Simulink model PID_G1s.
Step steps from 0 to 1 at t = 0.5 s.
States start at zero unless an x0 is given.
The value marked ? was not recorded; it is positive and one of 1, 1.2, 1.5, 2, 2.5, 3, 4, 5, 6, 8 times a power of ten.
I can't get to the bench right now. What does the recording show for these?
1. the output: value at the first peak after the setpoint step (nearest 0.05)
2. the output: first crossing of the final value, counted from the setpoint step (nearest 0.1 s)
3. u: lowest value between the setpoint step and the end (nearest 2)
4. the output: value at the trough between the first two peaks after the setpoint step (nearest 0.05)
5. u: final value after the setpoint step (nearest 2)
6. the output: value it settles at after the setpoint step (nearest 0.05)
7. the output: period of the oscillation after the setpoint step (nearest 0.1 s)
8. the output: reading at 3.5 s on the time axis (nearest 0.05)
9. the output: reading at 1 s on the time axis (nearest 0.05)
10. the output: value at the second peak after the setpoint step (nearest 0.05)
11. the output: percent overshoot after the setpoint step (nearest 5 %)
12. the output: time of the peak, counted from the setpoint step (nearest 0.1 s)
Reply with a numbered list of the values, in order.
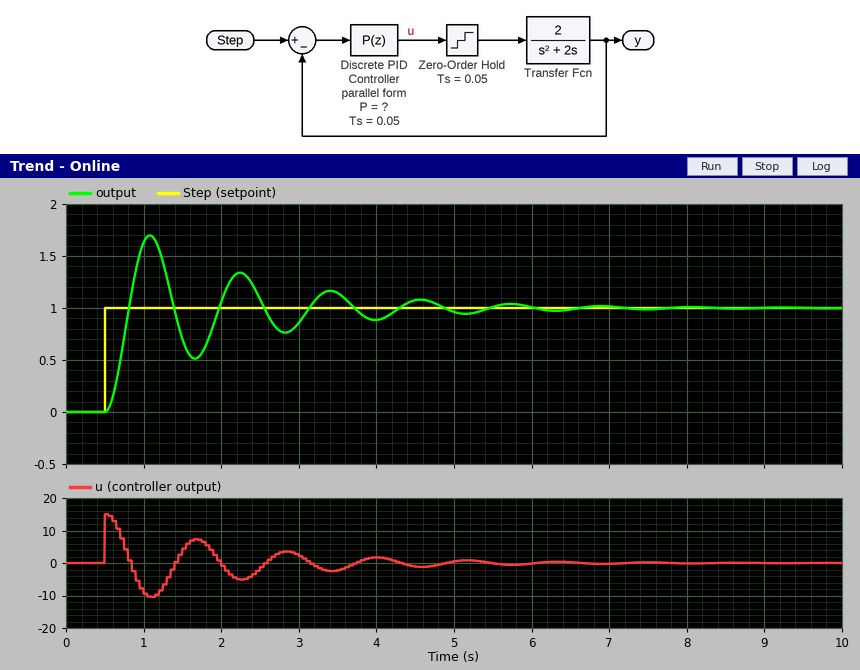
1. 1.70
2. 0.3 s
3. -10
4. 0.50
5. 0
6. 1.00
7. 1.2 s
8. 1.15
9. 1.65
10. 1.35
11. 70 %
12. 0.6 s
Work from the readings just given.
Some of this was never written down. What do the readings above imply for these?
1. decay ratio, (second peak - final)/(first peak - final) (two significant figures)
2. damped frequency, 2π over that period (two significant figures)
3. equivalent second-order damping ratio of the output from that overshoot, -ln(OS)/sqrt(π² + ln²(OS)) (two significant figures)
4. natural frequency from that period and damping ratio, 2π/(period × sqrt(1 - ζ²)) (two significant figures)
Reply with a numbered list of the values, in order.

1. 0.50
2. 5.2 rad/s
3. 0.11
4. 5.3 rad/s
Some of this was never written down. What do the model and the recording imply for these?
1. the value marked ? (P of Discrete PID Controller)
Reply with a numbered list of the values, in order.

1. 15
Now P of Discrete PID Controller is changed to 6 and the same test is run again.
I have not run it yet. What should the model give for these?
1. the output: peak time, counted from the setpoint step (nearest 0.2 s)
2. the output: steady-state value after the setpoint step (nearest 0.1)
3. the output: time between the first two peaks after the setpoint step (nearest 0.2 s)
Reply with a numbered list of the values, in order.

1. 1.0 s
2. 1.0
3. 1.8 s
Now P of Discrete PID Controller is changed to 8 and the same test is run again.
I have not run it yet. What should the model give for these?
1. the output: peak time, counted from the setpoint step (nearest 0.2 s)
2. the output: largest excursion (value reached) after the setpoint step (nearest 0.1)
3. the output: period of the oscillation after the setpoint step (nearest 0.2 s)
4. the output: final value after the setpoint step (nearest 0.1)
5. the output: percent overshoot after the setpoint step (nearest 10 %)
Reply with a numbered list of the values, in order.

1. 0.8 s
2. 1.5
3. 1.6 s
4. 1.0
5. 50 %
